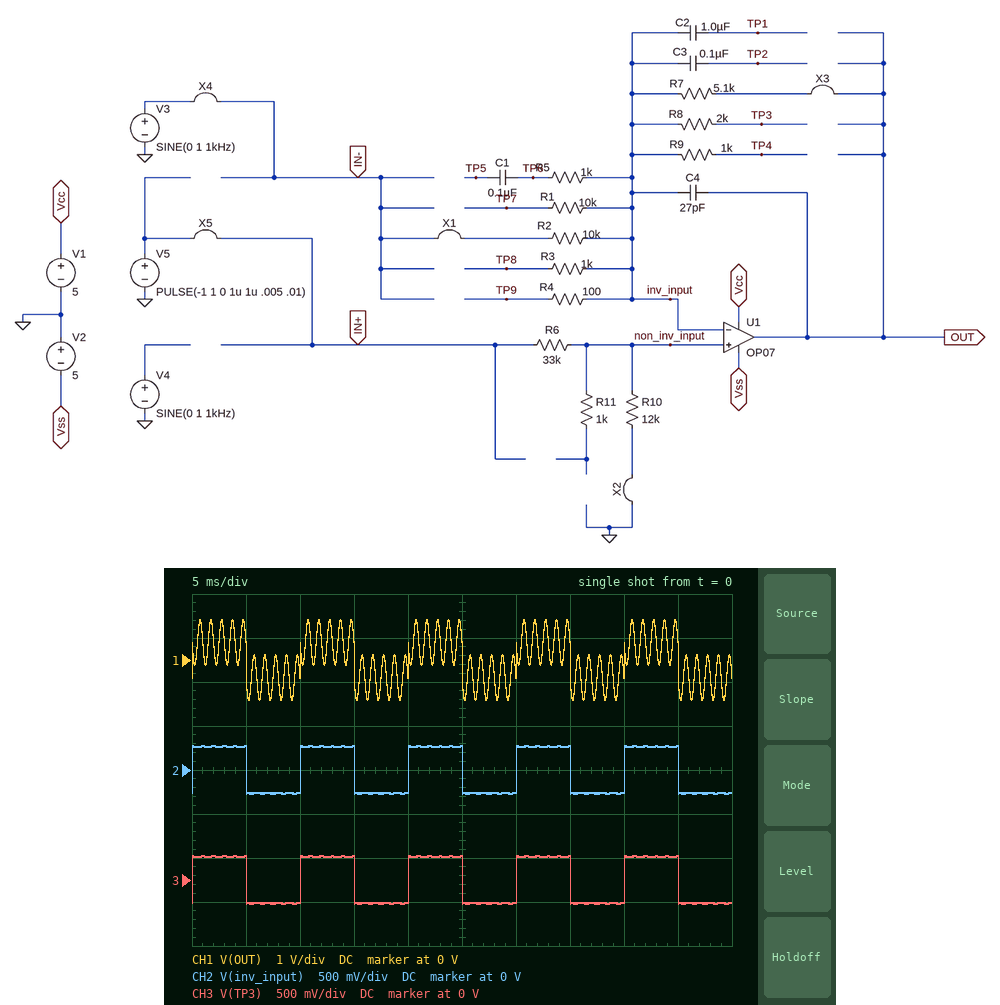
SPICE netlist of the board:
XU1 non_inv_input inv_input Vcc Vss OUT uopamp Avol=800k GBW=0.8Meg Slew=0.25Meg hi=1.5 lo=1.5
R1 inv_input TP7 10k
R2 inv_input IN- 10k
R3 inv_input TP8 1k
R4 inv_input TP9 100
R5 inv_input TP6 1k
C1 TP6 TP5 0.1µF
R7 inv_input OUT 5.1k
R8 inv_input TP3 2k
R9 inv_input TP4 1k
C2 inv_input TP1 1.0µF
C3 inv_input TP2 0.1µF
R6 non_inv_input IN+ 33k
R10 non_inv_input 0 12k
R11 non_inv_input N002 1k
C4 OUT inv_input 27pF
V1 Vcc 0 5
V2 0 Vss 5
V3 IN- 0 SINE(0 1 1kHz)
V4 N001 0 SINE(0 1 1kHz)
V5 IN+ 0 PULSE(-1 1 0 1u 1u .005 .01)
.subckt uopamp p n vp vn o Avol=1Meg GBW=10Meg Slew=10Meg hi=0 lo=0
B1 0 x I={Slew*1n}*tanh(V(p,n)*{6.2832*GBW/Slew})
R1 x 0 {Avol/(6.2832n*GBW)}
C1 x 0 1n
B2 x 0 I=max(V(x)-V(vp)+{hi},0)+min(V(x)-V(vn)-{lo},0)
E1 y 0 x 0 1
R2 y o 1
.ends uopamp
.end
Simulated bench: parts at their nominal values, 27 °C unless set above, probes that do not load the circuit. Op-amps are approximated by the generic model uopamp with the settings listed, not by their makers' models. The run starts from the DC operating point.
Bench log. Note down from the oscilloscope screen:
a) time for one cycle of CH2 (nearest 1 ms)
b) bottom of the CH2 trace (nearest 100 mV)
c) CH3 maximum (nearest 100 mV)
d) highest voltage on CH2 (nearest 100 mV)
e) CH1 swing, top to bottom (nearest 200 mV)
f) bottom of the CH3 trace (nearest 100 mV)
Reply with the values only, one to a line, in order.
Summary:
10 ms
-300 mV
300 mV
300 mV
1.8 V
-300 mV
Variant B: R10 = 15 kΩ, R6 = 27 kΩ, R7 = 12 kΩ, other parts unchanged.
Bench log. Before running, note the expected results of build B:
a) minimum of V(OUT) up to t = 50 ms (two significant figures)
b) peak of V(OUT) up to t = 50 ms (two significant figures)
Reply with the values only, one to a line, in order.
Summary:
-2.0 V
2.0 V
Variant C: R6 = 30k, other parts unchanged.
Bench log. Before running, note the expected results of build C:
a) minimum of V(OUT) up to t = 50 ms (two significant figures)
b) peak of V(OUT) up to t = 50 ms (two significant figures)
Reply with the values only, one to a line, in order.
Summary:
-940 mV
940 mV
